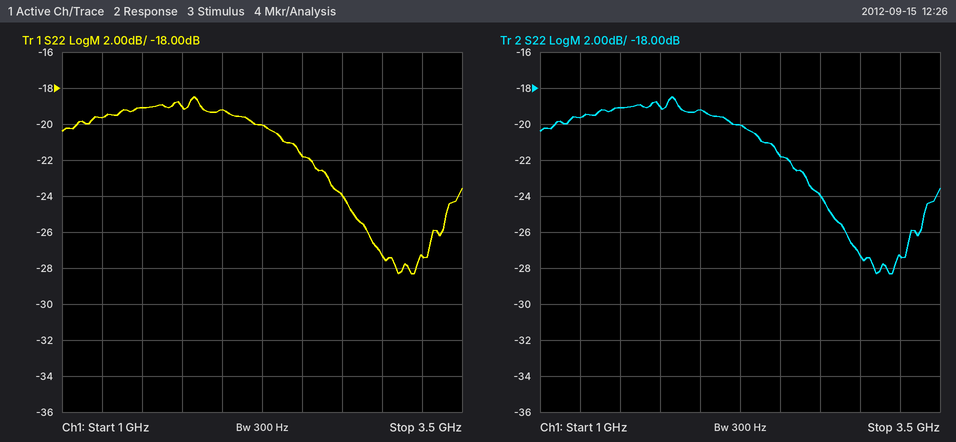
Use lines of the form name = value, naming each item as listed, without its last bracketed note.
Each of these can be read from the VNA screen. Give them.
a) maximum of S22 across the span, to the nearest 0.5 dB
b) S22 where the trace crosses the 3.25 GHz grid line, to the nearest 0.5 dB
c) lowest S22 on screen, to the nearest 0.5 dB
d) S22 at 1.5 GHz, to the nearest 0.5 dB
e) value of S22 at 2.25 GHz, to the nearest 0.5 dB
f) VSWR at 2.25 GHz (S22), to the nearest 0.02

maximum of S22 across the span, to the nearest 0.5 dB = -18.5 dB
S22 where the trace crosses the 3.25 GHz grid line, to the nearest 0.5 dB = -27.5 dB
lowest S22 on screen, to the nearest 0.5 dB = -28.5 dB
S22 at 1.5 GHz, to the nearest 0.5 dB = -19.0 dB
value of S22 at 2.25 GHz, to the nearest 0.5 dB = -20.0 dB
VSWR at 2.25 GHz (S22), to the nearest 0.02 = 1.22
